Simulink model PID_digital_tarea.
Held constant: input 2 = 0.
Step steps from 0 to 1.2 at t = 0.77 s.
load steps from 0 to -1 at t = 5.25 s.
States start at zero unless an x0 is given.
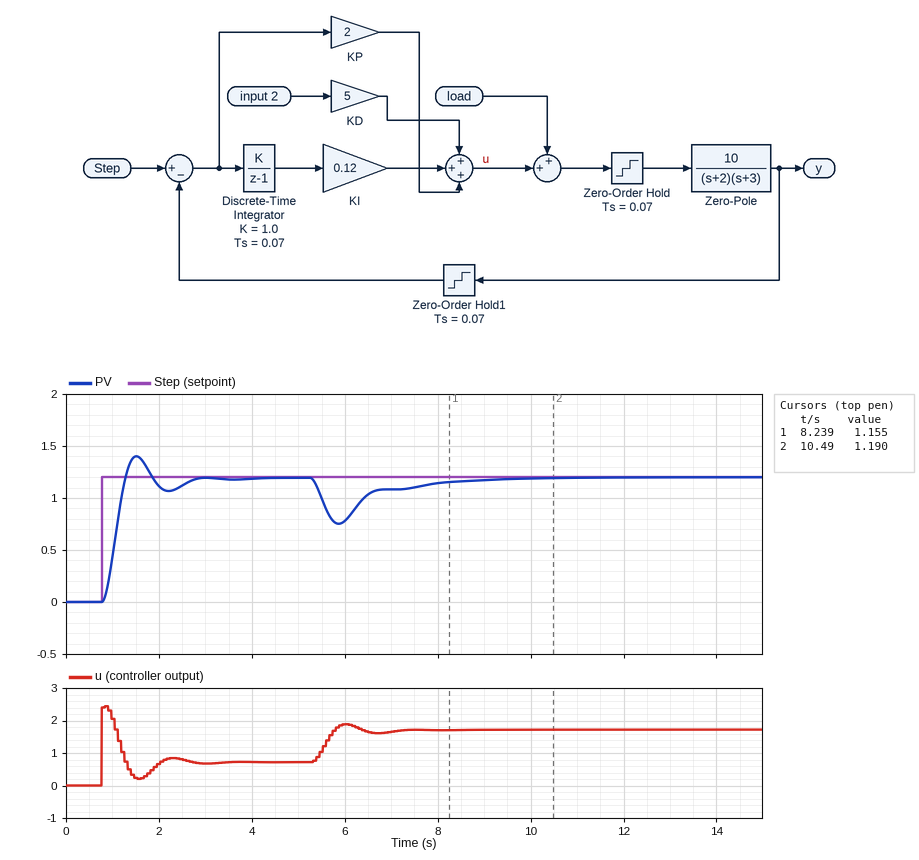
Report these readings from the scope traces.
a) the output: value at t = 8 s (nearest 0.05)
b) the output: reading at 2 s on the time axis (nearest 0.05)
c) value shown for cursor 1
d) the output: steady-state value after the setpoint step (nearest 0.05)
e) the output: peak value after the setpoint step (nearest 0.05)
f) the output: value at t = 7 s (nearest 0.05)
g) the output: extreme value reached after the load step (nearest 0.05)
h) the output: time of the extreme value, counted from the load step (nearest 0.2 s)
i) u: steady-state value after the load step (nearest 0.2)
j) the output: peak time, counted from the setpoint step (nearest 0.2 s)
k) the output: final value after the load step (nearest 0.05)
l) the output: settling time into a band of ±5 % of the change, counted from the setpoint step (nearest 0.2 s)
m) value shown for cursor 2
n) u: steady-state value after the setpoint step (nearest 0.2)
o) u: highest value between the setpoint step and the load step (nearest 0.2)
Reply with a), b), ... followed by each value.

a) 1.15
b) 1.10
c) 1.155
d) 1.20
e) 1.40
f) 1.10
g) 0.75
h) 0.6 s
i) 1.8
j) 0.8 s
k) 1.20
l) 1.8 s
m) 1.190
n) 0.8
o) 2.4
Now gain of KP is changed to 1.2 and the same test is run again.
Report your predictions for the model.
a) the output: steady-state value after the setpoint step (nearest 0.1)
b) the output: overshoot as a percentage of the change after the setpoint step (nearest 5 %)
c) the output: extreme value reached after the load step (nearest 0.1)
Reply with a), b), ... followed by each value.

a) 1.2
b) 15 %
c) 0.6
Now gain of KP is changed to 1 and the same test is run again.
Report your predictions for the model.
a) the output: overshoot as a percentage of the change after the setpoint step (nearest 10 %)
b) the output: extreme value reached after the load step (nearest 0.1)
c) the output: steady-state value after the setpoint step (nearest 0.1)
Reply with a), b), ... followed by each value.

a) 20 %
b) 0.6
c) 1.2
